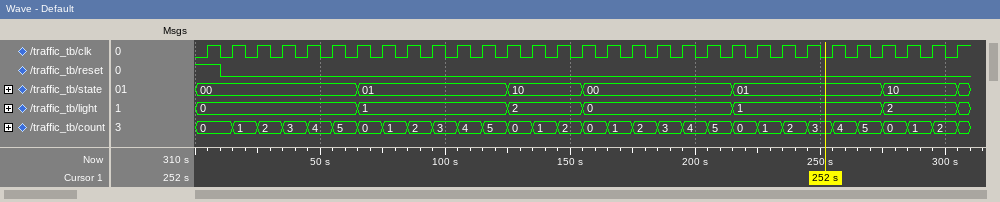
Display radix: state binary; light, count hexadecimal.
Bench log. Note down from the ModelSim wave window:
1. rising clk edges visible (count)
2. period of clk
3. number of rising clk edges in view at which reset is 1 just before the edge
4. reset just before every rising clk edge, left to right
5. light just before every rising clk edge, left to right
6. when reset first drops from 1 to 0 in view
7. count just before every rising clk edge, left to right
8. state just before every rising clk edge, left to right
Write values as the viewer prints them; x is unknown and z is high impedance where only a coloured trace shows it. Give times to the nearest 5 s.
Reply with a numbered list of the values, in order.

1. 31
2. 10 s
3. 1
4. 1 0 0 0 0 0 0 0 0 0 0 0 0 0 0 0 0 0 0 0 0 0 0 0 0 0 0 0 0 0 0
5. 0, 0, 0, 0, 0, 0, 0, 1, 1, 1, 1, 1, 1, 2, 2, 2, 0, 0, 0, 0, 0, 0, 1, 1, 1, 1, 1, 1, 2, 2, 2
6. 10 s
7. 0, 0, 1, 2, 3, 4, 5, 0, 1, 2, 3, 4, 5, 0, 1, 2, 0, 1, 2, 3, 4, 5, 0, 1, 2, 3, 4, 5, 0, 1, 2
8. 00, 00, 00, 00, 00, 00, 00, 01, 01, 01, 01, 01, 01, 10, 10, 10, 00, 00, 00, 00, 00, 00, 01, 01, 01, 01, 01, 01, 10, 10, 10
